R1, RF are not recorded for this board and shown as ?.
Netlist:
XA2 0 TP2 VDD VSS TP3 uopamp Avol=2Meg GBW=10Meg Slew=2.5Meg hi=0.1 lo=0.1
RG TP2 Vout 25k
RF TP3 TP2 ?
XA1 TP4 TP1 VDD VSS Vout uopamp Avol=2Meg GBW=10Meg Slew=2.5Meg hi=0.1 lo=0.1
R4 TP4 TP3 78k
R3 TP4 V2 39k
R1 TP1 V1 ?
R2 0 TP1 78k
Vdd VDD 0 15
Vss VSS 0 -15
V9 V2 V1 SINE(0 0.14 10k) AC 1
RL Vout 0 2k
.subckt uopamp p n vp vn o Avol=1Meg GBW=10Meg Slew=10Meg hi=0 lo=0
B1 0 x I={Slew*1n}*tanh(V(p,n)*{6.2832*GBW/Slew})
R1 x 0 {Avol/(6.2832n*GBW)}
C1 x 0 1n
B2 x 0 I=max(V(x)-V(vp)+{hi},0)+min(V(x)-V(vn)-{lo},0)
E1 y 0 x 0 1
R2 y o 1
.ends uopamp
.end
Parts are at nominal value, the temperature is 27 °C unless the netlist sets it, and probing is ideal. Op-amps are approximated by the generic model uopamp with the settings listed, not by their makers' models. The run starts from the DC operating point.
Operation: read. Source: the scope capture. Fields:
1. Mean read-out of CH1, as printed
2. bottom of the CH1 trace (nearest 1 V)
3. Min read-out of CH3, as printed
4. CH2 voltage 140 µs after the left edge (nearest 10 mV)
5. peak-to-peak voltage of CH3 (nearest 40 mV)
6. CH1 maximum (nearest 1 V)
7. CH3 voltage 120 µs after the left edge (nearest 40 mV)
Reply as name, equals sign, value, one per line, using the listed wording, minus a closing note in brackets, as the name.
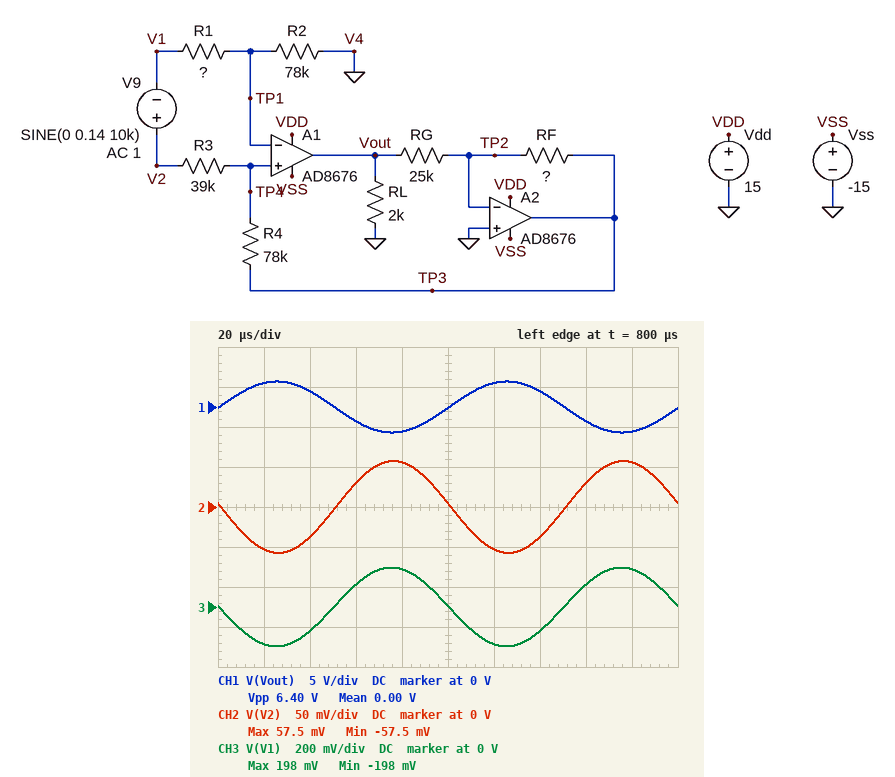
Mean read-out of CH1, as printed = 0.00 V
bottom of the CH1 trace = -3 V
Min read-out of CH3, as printed = -198 mV
CH2 voltage 140 µs after the left edge = -40 mV
peak-to-peak voltage of CH3 = 400 mV
CH1 maximum = 3 V
CH3 voltage 120 µs after the left edge = -200 mV
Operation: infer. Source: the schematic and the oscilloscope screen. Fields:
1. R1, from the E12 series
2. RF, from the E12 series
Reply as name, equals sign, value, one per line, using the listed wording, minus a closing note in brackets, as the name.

R1, from the E12 series = 56 kΩ
RF, from the E12 series = 1.8 kΩ
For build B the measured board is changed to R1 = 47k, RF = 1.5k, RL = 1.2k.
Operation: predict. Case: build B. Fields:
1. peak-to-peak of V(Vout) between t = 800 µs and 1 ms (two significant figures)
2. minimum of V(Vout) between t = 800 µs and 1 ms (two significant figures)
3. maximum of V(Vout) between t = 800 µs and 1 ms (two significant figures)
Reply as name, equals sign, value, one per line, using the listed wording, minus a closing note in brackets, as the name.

peak-to-peak of V(Vout) between t = 800 µs and 1 ms = 8.5 V
minimum of V(Vout) between t = 800 µs and 1 ms = -4.2 V
maximum of V(Vout) between t = 800 µs and 1 ms = 4.2 V
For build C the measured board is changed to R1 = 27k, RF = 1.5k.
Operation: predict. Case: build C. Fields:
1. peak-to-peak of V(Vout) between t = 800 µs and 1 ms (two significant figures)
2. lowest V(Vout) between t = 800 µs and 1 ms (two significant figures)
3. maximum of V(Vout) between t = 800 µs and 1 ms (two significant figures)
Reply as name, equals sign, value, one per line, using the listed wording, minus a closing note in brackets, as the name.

peak-to-peak of V(Vout) between t = 800 µs and 1 ms = 11 V
lowest V(Vout) between t = 800 µs and 1 ms = -5.5 V
maximum of V(Vout) between t = 800 µs and 1 ms = 5.5 V
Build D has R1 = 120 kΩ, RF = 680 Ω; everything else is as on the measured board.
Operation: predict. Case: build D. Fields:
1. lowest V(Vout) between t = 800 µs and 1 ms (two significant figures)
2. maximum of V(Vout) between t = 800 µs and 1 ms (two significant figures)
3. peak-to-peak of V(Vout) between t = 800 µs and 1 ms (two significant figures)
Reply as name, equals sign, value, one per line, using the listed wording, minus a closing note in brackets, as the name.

lowest V(Vout) between t = 800 µs and 1 ms = -5.0 V
maximum of V(Vout) between t = 800 µs and 1 ms = 5.0 V
peak-to-peak of V(Vout) between t = 800 µs and 1 ms = 10 V
